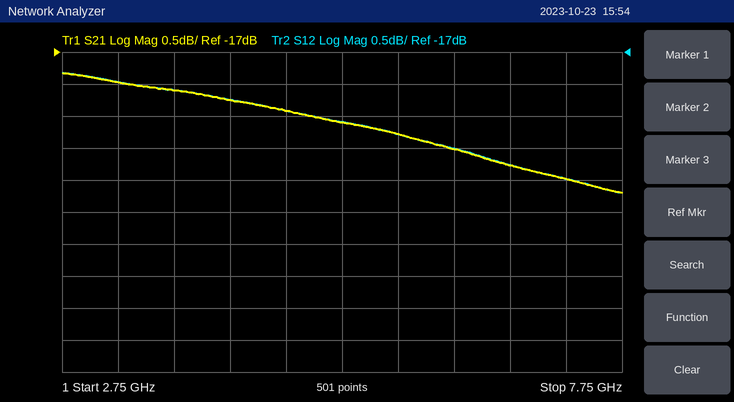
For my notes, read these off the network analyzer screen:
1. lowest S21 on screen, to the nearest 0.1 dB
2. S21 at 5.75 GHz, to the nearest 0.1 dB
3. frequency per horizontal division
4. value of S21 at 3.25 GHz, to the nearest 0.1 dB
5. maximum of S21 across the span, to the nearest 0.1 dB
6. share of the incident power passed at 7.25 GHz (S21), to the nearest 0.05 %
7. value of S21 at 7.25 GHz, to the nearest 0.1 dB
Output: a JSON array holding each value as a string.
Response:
["-19.2 dB", "-18.3 dB", "500 MHz", "-17.5 dB", "-17.3 dB", "1.25 %", "-19.0 dB"]
